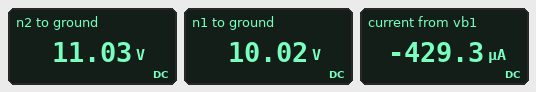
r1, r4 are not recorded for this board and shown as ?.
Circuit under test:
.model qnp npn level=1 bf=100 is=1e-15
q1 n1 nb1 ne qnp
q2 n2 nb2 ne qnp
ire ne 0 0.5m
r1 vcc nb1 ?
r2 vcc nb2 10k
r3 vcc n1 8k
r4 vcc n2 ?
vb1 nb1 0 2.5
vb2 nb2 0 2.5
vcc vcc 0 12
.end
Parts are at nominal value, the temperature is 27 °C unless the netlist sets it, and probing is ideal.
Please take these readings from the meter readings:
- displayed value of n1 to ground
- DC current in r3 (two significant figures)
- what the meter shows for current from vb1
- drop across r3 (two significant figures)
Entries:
10.02 V
250 µA
-429.3 µA
2.0 V
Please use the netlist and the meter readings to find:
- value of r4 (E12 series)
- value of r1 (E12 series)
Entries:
3.9 kΩ
22 kΩ
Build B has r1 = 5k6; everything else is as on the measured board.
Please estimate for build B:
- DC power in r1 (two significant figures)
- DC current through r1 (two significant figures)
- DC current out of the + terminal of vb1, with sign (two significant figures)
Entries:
16 mW
1.7 mA
-1.7 mA
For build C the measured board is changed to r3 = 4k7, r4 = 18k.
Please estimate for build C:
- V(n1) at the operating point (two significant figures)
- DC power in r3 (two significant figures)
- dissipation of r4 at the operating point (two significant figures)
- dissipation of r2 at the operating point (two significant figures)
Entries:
11 V
290 µW
1.1 mW
9.0 mW
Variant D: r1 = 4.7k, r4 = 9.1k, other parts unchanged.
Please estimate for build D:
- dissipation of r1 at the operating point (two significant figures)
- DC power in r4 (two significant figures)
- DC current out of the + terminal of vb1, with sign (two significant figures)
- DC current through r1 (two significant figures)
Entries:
19 mW
560 µW
-2.0 mA
2.0 mA
